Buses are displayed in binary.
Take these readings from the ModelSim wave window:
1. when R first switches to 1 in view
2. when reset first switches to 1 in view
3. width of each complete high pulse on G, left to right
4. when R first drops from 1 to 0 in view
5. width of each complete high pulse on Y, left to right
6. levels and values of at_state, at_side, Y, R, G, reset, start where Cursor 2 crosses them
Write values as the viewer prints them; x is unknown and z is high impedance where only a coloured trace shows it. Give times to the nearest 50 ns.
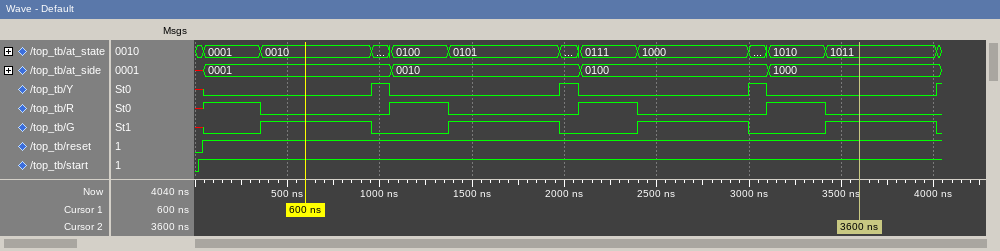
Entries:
50 ns
50 ns
600 ns, 600 ns, 600 ns, 600 ns
350 ns
100 ns, 100 ns, 100 ns
at_state=1011, at_side=1000, Y=0, R=0, G=1, reset=1, start=1
